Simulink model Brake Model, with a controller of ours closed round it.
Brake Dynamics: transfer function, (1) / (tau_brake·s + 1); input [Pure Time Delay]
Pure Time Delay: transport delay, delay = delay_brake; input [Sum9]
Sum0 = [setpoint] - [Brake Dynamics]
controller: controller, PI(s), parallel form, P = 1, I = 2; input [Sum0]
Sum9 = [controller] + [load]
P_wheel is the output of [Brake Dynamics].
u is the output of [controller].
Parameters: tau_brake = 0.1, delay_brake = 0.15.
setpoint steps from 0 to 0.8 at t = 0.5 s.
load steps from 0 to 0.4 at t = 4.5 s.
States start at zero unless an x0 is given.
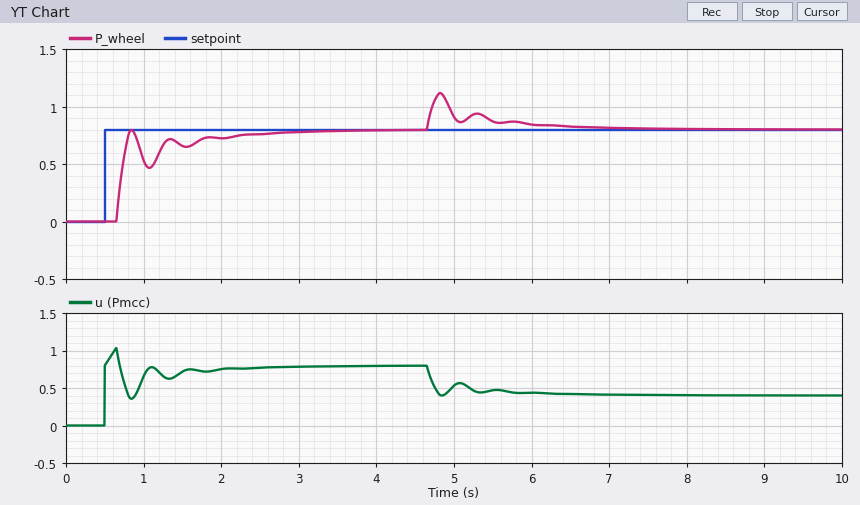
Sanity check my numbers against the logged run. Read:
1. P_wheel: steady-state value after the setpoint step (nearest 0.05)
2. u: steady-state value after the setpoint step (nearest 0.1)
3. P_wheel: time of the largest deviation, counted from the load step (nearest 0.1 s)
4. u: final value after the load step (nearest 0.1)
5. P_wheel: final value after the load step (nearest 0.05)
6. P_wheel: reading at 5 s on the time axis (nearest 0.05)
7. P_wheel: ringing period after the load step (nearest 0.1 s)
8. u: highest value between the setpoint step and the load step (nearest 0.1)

0.80
0.8
0.3 s
0.4
0.80
0.90
0.5 s
1.0
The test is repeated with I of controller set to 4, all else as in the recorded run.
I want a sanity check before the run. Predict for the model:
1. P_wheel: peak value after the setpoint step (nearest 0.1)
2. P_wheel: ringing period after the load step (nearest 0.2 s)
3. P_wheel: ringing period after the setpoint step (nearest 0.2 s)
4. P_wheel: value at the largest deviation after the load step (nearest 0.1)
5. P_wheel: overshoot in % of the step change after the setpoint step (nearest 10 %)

1.0
0.6 s
0.6 s
1.1
20 %
